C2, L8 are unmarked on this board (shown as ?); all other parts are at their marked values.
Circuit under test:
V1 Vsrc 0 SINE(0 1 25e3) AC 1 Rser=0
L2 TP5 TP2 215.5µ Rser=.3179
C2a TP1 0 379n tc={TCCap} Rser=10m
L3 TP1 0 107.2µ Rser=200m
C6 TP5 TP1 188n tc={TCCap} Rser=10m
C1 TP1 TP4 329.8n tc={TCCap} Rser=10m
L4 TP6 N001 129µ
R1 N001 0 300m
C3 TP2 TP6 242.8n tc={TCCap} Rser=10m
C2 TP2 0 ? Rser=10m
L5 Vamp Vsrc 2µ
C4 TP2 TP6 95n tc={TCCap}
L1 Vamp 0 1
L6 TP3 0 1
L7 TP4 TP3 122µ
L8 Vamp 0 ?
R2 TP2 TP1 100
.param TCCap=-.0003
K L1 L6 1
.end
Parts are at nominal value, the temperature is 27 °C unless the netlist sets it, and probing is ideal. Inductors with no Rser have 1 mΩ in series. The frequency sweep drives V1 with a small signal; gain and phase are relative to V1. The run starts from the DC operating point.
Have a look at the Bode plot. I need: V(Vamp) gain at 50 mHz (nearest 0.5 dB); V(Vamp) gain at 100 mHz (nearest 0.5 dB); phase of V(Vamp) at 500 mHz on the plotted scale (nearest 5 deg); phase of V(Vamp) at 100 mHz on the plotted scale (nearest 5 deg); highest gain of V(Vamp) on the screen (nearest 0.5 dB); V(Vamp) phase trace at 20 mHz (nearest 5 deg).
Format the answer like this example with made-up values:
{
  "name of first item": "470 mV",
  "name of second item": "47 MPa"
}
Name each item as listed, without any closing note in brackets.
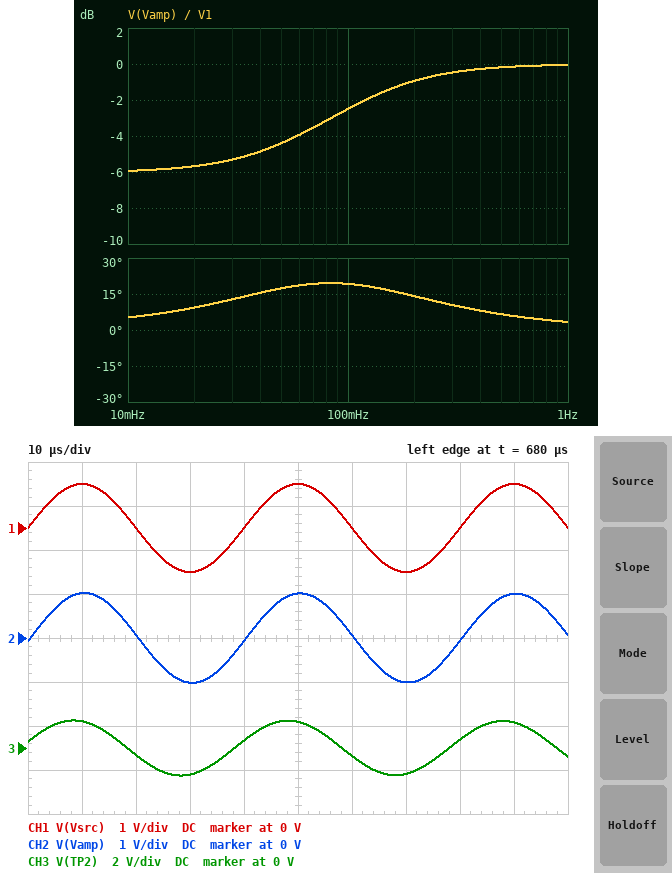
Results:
{
  "V(Vamp) gain at 50 mHz": "-4.5 dB",
  "V(Vamp) gain at 100 mHz": "-2.5 dB",
  "phase of V(Vamp) at 500 mHz on the plotted scale": "5 deg",
  "phase of V(Vamp) at 100 mHz on the plotted scale": "20 deg",
  "highest gain of V(Vamp) on the screen": "0 dB",
  "V(Vamp) phase trace at 20 mHz": "10 deg"
}
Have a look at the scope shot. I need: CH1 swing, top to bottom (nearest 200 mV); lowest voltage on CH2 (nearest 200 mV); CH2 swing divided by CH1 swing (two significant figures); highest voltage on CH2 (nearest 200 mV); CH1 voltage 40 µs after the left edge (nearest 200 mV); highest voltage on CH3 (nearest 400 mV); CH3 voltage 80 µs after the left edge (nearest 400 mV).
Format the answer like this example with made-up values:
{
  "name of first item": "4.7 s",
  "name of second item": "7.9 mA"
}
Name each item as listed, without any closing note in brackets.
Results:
{
  "CH1 swing, top to bottom": "2.0 V",
  "lowest voltage on CH2": "-1.0 V",
  "CH2 swing divided by CH1 swing": "1.0",
  "highest voltage on CH2": "1.0 V",
  "CH1 voltage 40 µs after the left edge": "0 V",
  "highest voltage on CH3": "1.2 V",
  "CH3 voltage 80 µs after the left edge": "400 mV"
}
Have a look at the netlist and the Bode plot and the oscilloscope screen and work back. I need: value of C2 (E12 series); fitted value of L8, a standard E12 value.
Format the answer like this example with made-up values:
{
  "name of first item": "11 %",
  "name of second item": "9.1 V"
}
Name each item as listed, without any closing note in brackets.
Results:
{
  "value of C2": "3.9 µF",
  "fitted value of L8, a standard E12 value": "2.7 mH"
}
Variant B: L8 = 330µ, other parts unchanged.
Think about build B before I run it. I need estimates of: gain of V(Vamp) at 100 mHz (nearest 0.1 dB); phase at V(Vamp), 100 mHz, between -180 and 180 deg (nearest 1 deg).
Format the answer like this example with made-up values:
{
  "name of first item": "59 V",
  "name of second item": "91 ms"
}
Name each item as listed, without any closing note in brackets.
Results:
{
  "gain of V(Vamp) at 100 mHz": "-5.9 dB",
  "phase at V(Vamp), 100 mHz, between -180 and 180 deg": "6 deg"
}
